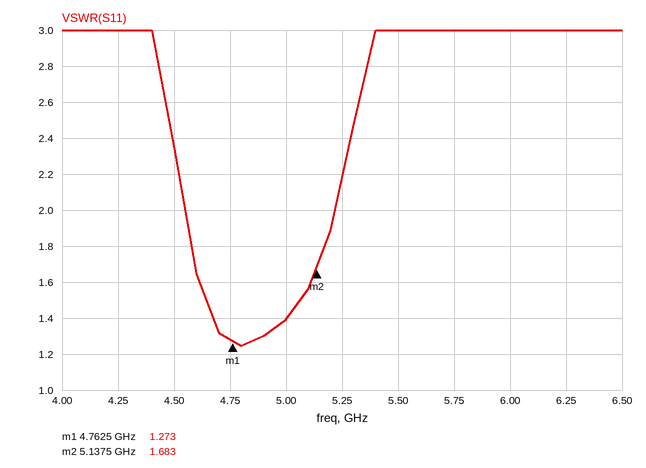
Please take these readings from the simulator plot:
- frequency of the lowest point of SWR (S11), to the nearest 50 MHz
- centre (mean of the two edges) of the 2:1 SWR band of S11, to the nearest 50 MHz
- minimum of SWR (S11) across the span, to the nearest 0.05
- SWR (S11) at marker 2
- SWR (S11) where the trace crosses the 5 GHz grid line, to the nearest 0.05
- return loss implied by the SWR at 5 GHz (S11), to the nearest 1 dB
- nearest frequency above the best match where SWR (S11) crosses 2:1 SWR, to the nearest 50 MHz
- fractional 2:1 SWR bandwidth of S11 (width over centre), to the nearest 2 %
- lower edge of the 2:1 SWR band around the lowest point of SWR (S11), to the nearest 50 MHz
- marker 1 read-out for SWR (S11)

4.80 GHz
4.90 GHz
1.25
1.683
1.40
16 dB
5.20 GHz
14 %
4.55 GHz
1.273
